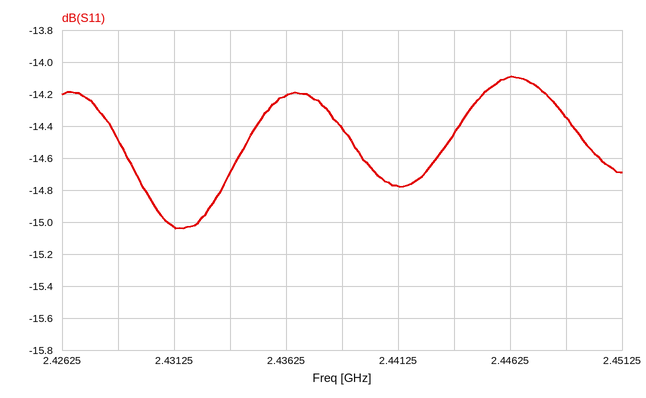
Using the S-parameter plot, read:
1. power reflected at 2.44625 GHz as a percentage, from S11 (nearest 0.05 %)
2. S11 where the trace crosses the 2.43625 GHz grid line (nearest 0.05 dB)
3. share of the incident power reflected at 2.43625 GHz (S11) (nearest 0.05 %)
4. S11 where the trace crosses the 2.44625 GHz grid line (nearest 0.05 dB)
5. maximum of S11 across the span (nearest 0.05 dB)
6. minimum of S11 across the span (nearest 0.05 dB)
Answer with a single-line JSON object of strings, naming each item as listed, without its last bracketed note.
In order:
{"power reflected at 2.44625 GHz as a percentage, from S11": "3.90 %", "S11 where the trace crosses the 2.43625 GHz grid line": "-14.20 dB", "share of the incident power reflected at 2.43625 GHz (S11)": "3.80 %", "S11 where the trace crosses the 2.44625 GHz grid line": "-14.10 dB", "maximum of S11 across the span": "-14.10 dB", "minimum of S11 across the span": "-15.05 dB"}
